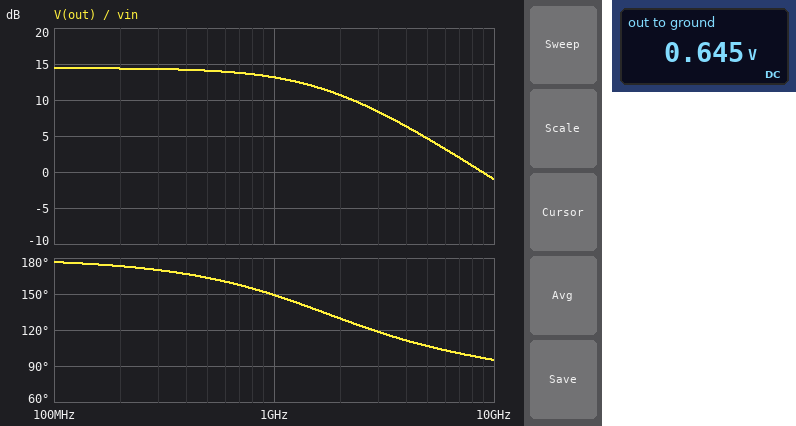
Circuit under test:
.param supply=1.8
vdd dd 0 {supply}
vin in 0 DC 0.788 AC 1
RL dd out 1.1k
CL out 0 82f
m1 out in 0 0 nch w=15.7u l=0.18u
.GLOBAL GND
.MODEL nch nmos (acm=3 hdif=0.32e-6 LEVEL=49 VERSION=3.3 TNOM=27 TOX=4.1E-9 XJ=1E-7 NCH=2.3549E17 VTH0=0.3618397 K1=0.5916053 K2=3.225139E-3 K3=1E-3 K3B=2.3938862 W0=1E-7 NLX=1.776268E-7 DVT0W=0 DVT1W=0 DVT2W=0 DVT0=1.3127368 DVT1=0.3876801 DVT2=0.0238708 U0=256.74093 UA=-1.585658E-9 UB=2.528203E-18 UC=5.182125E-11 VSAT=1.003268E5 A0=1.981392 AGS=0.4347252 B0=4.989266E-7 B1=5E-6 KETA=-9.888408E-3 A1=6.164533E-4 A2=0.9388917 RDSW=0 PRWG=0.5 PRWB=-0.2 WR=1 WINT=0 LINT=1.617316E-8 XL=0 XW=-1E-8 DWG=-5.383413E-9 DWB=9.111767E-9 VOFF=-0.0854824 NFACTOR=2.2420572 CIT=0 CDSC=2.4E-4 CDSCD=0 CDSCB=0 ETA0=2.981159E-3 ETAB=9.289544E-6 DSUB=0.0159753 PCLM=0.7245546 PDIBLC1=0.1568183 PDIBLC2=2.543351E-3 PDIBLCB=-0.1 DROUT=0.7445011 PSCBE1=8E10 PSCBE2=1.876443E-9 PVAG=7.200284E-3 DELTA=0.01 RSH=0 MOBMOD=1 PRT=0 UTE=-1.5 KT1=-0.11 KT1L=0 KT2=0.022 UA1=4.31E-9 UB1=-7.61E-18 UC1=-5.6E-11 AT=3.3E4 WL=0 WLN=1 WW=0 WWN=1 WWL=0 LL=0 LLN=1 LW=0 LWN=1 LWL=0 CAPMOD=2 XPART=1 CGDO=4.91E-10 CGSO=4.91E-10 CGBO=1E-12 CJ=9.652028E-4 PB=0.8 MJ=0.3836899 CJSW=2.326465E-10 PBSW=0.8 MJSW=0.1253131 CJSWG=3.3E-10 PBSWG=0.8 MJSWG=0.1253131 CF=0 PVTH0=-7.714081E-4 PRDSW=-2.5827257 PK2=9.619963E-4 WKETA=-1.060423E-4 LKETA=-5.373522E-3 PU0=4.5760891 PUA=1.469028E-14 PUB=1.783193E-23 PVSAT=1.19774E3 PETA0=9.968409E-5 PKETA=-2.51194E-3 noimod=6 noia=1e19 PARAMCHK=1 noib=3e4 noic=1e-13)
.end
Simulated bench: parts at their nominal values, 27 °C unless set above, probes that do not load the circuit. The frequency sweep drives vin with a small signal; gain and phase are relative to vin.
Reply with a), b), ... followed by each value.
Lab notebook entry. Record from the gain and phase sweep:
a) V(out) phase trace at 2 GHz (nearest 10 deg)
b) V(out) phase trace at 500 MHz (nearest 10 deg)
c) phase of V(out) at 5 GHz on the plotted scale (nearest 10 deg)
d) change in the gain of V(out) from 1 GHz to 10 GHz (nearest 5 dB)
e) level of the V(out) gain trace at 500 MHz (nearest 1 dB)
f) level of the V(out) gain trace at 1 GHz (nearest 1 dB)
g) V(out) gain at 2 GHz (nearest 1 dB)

a) 130 deg
b) 160 deg
c) 110 deg
d) -15 dB
e) 14 dB
f) 13 dB
g) 11 dB
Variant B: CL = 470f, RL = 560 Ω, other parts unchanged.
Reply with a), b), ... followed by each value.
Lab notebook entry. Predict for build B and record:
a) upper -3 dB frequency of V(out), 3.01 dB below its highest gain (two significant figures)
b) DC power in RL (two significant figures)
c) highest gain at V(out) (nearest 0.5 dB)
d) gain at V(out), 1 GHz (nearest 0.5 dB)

a) 640 MHz
b) 750 µW
c) 10.0 dB
d) 4.5 dB
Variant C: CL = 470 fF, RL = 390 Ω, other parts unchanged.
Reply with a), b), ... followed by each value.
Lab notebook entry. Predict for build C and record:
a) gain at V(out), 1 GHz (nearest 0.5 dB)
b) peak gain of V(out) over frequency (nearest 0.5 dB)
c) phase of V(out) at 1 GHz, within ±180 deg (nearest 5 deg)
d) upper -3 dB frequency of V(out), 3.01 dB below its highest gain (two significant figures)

a) 4.0 dB
b) 7.5 dB
c) 130 deg
d) 890 MHz
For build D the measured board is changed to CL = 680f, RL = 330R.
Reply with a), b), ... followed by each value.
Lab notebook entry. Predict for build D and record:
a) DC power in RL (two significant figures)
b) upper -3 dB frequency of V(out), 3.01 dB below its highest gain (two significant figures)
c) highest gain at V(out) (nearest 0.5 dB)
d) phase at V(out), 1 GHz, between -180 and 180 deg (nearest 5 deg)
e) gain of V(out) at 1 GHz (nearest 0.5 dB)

a) 480 µW
b) 730 MHz
c) 6.0 dB
d) 125 deg
e) 1.5 dB
